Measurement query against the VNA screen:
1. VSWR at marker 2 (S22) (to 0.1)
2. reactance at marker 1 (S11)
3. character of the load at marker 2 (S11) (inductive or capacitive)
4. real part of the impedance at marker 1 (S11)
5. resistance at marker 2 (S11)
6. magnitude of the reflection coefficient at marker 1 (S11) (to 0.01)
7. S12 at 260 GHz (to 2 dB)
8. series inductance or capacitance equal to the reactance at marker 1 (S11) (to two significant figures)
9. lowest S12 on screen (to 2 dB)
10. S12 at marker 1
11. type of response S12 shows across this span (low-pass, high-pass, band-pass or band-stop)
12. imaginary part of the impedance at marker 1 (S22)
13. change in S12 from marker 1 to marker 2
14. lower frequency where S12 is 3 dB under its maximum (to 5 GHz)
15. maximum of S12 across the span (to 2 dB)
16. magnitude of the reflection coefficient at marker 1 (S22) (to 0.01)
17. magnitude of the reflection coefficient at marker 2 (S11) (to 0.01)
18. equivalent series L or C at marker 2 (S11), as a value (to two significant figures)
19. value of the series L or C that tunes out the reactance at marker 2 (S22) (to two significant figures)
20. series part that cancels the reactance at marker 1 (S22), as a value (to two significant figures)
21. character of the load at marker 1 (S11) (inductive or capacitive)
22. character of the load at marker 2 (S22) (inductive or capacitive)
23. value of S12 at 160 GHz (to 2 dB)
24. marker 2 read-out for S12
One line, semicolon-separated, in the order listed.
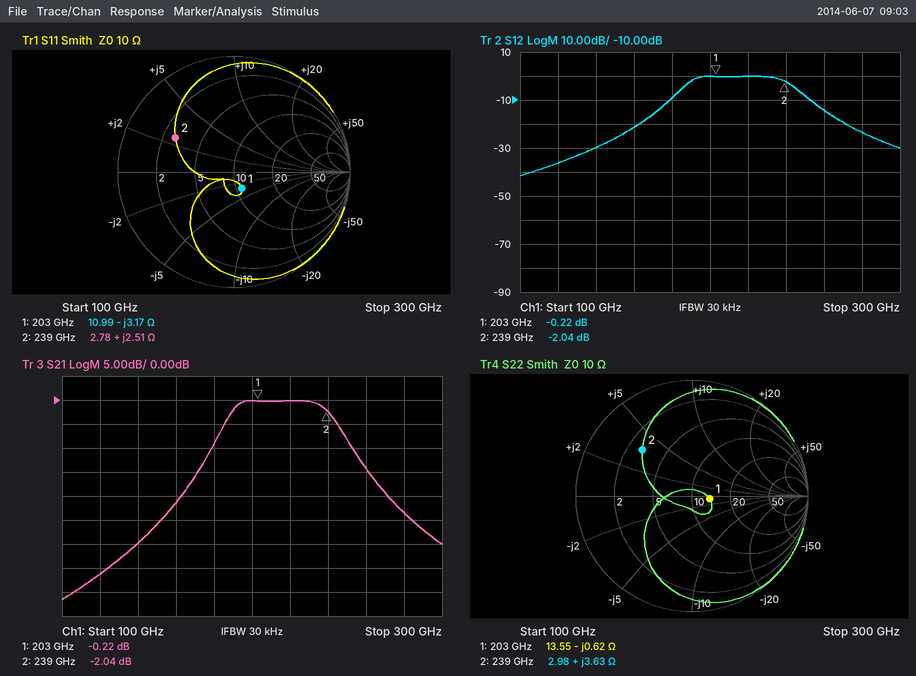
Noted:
3.8; -3.17 Ω; inductive; 10.99 Ω; 2.78 Ω; 0.16; -14 dB; 250 fF; -42 dB; -0.22 dB; band-pass; -0.62 Ω; -1.82 dB; 190 GHz; 0 dB; 0.15; 0.59; 1.7 pH; 180 fF; 490 fH; capacitive; inductive; -22 dB; -2.04 dB
